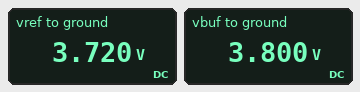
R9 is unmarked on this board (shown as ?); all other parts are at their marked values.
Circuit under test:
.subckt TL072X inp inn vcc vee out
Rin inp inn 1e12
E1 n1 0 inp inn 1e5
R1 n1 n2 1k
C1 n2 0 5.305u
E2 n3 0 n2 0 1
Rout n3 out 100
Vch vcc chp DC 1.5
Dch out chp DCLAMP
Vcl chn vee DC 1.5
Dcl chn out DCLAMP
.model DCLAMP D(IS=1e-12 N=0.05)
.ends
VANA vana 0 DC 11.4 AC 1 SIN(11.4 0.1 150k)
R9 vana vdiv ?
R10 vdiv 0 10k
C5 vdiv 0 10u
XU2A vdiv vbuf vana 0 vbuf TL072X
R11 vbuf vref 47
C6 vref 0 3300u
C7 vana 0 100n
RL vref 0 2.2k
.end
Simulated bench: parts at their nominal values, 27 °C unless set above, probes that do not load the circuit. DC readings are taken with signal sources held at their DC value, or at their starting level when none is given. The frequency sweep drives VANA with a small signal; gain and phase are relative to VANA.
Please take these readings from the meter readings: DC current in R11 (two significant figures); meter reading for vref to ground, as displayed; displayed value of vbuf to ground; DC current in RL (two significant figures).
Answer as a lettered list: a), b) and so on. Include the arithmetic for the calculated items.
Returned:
a) (3.8 V - 3.72 V) / 47 Ω = 1.7 mA
b) 3.720 V
c) 3.800 V
d) (3.72 V) / 2.2 kΩ = 1.7 mA
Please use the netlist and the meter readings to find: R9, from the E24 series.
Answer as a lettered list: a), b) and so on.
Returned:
a) 20 kΩ
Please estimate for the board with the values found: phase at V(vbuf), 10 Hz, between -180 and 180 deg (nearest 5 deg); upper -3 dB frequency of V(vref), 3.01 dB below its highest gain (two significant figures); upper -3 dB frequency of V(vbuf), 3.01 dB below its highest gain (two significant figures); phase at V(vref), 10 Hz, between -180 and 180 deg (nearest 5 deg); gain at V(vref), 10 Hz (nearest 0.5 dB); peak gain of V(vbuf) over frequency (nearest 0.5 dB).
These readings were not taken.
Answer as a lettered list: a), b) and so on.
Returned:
a) -75 deg
b) 910 mHz
c) 2.4 Hz
d) -160 deg
e) -42.0 dB
f) -9.5 dB
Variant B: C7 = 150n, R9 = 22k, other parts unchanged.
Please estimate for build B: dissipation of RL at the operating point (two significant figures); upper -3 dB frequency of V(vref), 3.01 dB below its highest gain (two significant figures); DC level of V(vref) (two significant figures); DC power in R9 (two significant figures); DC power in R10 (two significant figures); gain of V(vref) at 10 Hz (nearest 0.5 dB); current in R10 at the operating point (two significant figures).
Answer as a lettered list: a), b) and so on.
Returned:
a) 5.5 mW
b) 900 mHz
c) 3.5 V
d) 2.8 mW
e) 1.3 mW
f) -43.0 dB
g) 360 µA
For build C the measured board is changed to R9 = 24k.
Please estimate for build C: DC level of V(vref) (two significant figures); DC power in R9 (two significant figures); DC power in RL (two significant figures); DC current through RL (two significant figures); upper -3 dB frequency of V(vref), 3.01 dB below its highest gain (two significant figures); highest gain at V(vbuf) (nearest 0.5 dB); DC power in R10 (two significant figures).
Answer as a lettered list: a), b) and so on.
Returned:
a) 3.3 V
b) 2.7 mW
c) 4.9 mW
d) 1.5 mA
e) 890 mHz
f) -10.5 dB
g) 1.1 mW
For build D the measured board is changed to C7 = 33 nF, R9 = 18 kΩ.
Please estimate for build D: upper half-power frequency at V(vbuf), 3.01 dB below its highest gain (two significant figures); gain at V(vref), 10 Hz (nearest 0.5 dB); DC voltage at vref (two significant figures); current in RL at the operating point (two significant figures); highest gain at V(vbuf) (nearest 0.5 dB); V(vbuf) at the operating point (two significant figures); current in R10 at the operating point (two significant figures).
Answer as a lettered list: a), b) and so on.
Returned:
a) 2.5 Hz
b) -41.0 dB
c) 4.0 V
d) 1.8 mA
e) -9.0 dB
f) 4.1 V
g) 410 µA
